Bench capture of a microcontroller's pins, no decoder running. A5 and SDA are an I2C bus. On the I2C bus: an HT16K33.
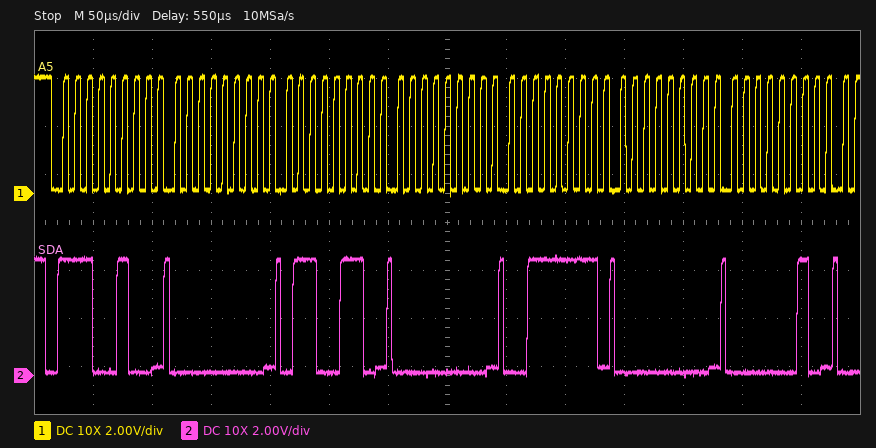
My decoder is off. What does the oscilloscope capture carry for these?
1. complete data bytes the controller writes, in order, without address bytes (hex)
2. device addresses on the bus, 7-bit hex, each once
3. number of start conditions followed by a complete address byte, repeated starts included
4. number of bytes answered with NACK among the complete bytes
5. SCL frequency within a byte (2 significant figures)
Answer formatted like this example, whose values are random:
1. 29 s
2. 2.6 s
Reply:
1. 00 66 00 3F 00 02
2. 0x72
3. 1
4. 0
5. 100 kHz
